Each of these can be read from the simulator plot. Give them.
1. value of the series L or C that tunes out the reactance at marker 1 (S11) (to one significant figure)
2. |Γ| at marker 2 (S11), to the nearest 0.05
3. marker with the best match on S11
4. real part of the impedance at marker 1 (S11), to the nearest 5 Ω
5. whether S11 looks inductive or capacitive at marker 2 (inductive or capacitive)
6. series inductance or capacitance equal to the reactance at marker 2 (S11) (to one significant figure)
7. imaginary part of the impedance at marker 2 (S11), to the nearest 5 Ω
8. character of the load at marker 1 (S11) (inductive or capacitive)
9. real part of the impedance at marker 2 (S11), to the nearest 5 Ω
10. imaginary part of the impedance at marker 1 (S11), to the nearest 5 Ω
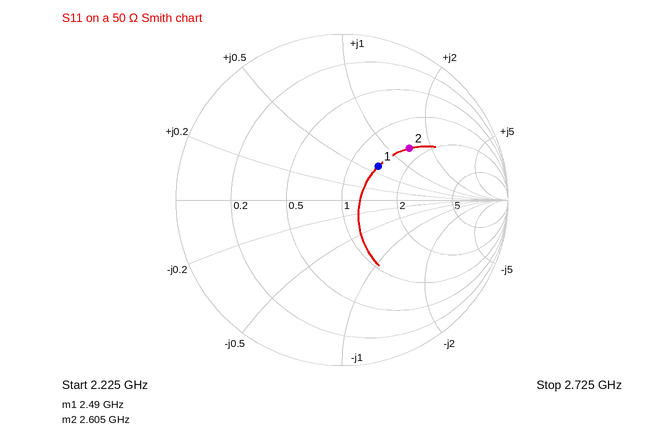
2 pF
0.50
marker 1
70 Ω
inductive
4 nH
+70 Ω
inductive
80 Ω
+30 Ω
